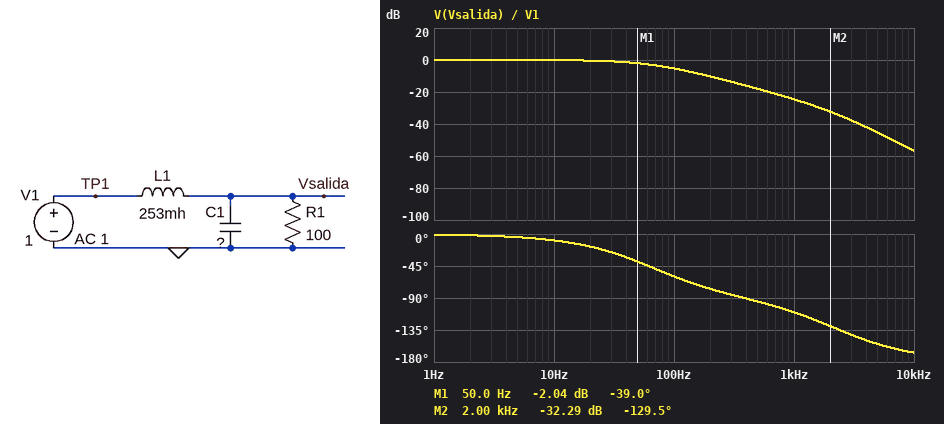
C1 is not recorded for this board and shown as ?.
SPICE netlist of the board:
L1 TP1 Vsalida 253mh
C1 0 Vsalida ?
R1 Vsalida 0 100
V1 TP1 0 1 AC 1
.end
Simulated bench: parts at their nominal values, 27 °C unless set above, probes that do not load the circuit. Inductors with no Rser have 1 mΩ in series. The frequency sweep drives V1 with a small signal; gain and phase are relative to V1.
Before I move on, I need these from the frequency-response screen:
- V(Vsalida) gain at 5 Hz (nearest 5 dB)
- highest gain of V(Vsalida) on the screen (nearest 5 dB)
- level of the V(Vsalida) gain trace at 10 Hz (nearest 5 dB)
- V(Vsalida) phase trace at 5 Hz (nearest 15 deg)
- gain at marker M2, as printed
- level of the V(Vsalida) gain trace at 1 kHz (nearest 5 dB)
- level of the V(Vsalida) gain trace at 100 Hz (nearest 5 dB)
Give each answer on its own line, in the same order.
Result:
0 dB
0 dB
0 dB
0 deg
-32.29 dB
-25 dB
-5 dB
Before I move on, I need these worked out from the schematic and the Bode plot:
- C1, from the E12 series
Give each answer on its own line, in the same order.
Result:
680 nF
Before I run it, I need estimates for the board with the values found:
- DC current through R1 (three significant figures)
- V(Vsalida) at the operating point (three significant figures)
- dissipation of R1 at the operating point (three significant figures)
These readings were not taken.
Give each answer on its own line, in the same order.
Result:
10.0 mA
1.00 V
10.0 mW
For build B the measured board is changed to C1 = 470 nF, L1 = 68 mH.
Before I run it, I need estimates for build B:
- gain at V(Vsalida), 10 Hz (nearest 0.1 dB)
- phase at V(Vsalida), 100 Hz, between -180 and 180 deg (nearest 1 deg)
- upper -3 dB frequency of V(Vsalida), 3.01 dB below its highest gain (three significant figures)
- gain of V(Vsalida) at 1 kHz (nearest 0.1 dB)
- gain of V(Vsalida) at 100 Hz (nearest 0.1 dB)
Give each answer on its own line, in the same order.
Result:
0 dB
-23 deg
251 Hz
-12.6 dB
-0.6 dB
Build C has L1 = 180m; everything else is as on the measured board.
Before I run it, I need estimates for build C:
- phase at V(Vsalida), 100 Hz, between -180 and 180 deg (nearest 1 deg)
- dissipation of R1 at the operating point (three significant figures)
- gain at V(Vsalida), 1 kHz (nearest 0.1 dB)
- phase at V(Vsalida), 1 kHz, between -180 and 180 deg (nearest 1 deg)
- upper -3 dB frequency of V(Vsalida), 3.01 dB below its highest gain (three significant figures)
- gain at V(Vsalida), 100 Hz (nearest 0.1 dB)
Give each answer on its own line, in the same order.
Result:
-50 deg
10.0 mW
-21.5 dB
-109 deg
91.9 Hz
-3.4 dB
